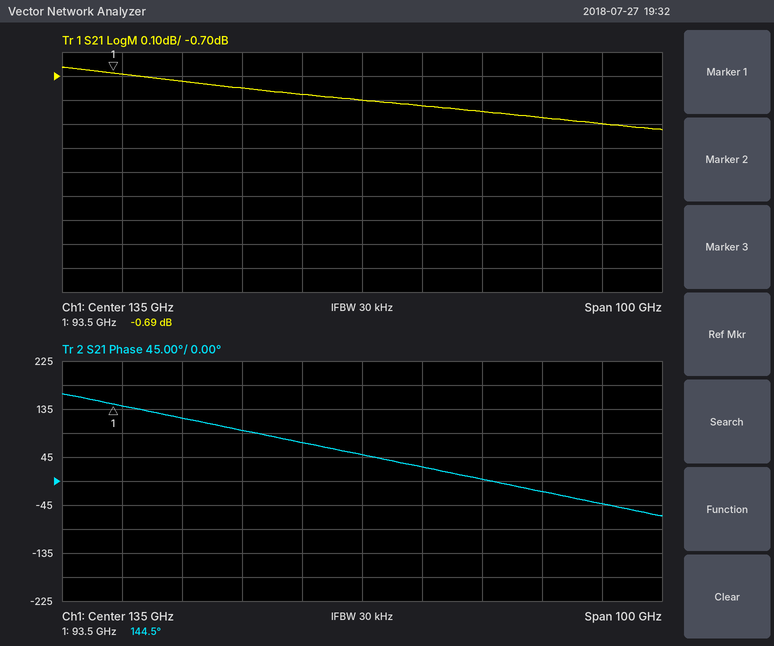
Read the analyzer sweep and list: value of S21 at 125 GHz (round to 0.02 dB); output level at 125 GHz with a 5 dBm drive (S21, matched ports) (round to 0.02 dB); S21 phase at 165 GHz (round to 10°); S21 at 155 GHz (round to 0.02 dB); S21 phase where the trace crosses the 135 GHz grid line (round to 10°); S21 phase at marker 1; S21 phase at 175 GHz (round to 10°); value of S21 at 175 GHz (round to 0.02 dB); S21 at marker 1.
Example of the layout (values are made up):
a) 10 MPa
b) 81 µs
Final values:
a) -0.78 dB
b) 4.22 dBm
c) -20°
d) -0.84 dB
e) 50°
f) 144.5°
g) -40°
h) -0.90 dB
i) -0.69 dB
